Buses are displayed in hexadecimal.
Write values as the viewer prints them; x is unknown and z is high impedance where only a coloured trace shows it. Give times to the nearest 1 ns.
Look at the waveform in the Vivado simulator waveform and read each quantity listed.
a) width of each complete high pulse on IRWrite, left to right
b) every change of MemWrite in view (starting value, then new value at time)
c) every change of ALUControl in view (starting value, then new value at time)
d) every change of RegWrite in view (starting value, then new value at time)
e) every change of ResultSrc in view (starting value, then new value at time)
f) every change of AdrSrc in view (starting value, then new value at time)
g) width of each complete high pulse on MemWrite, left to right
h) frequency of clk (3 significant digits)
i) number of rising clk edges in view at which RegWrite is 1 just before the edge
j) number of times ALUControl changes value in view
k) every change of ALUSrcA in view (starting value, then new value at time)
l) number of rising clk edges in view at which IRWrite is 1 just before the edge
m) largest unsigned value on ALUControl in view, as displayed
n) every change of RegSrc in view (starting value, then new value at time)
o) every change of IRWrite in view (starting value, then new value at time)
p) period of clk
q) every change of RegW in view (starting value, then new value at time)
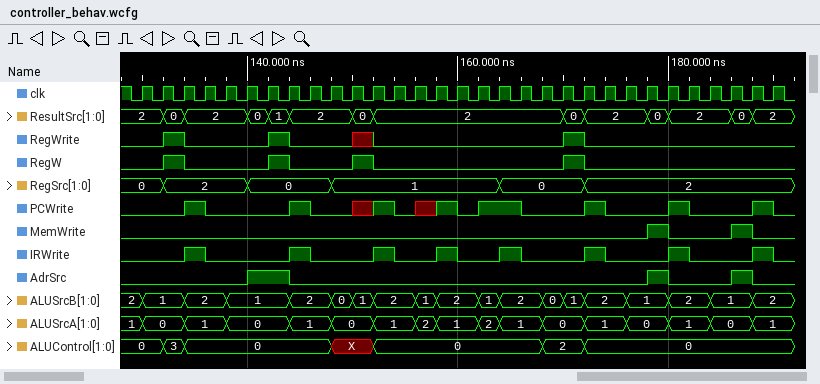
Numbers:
2 ns, 2 ns, 2 ns, 2 ns, 2 ns, 2 ns, 2 ns, 2 ns
0, 1 at 178 ns, 0 at 180 ns, 1 at 186 ns, 0 at 188 ns
0, 3 at 132 ns, 0 at 134 ns, X at 148 ns, 0 at 152 ns, 2 at 168 ns, 0 at 172 ns
0, 1 at 132 ns, 0 at 134 ns, 1 at 142 ns, 0 at 144 ns, x at 150 ns, 0 at 152 ns, 1 at 170 ns, 0 at 172 ns
2, 0 at 132 ns, 2 at 134 ns, 0 at 140 ns, 1 at 142 ns, 2 at 144 ns, 0 at 150 ns, 2 at 152 ns, 0 at 170 ns, 2 at 172 ns, 0 at 178 ns, 2 at 180 ns, 0 at 186 ns, 2 at 188 ns
0, 1 at 140 ns, 0 at 144 ns, 1 at 178 ns, 0 at 180 ns, 1 at 186 ns, 0 at 188 ns
2 ns, 2 ns
500 MHz
3
6
1, 0 at 130 ns, 1 at 134 ns, 0 at 138 ns, 1 at 144 ns, 0 at 148 ns, 1 at 152 ns, 2 at 156 ns, 1 at 158 ns, 2 at 162 ns, 1 at 164 ns, 0 at 168 ns, 1 at 172 ns, 0 at 176 ns, 1 at 180 ns, 0 at 184 ns, 1 at 188 ns
8
3
0, 2 at 132 ns, 0 at 140 ns, 1 at 148 ns, 0 at 164 ns, 2 at 172 ns
0, 1 at 134 ns, 0 at 136 ns, 1 at 144 ns, 0 at 146 ns, 1 at 152 ns, 0 at 154 ns, 1 at 158 ns, 0 at 160 ns, 1 at 164 ns, 0 at 166 ns, 1 at 172 ns, 0 at 174 ns, 1 at 180 ns, 0 at 182 ns, 1 at 188 ns, 0 at 190 ns
2 ns
0, 1 at 132 ns, 0 at 134 ns, 1 at 142 ns, 0 at 144 ns, 1 at 150 ns, 0 at 152 ns, 1 at 170 ns, 0 at 172 ns
